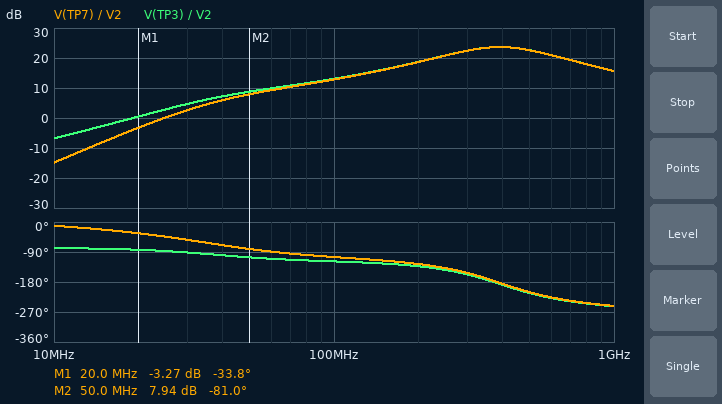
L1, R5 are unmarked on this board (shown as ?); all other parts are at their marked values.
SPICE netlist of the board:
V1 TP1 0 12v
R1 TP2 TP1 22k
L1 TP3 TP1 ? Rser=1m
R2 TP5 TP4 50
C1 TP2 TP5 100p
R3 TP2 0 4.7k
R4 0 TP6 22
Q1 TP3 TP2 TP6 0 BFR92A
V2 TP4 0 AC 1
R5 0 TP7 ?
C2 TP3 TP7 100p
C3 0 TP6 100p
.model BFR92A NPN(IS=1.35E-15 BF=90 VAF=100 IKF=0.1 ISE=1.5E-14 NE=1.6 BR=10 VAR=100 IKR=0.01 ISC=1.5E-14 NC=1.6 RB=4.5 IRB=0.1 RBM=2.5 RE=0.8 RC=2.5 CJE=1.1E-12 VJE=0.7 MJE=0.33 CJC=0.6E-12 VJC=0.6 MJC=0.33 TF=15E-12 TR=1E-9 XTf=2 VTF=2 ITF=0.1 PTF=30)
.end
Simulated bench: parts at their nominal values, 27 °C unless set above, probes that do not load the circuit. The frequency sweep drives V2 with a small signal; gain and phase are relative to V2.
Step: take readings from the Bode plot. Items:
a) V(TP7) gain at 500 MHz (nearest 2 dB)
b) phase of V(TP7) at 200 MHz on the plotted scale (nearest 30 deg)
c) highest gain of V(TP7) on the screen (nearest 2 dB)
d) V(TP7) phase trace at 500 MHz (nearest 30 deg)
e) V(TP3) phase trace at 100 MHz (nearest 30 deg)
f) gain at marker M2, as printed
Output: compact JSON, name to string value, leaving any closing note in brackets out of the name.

{"V(TP7) gain at 500 MHz": "22 dB", "phase of V(TP7) at 200 MHz on the plotted scale": "-120 deg", "highest gain of V(TP7) on the screen": "24 dB", "V(TP7) phase trace at 500 MHz": "-210 deg", "V(TP3) phase trace at 100 MHz": "-120 deg", "gain at marker M2, as printed": "7.94 dB"}
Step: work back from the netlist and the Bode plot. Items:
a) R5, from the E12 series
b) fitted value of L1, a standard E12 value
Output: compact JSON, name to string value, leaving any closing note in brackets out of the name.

{"R5, from the E12 series": "68 Ω", "fitted value of L1, a standard E12 value": "180 nH"}
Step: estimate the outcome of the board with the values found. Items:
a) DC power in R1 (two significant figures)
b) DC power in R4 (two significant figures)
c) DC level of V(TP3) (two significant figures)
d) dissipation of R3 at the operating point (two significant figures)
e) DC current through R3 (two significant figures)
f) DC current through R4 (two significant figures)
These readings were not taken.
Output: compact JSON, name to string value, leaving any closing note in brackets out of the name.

{"DC power in R1": "5.3 mW", "DC power in R4": "8.2 mW", "DC level of V(TP3)": "12 V", "dissipation of R3 at the operating point": "320 µW", "DC current through R3": "260 µA", "DC current through R4": "19 mA"}
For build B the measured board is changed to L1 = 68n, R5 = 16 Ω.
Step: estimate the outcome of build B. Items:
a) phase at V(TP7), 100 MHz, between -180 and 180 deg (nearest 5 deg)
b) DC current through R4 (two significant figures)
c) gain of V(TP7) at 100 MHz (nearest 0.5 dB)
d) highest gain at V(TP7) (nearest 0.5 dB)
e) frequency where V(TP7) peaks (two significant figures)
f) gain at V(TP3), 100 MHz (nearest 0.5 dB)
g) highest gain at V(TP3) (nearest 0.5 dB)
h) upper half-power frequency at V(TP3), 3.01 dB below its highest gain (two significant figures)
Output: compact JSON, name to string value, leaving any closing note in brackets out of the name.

{"phase at V(TP7), 100 MHz, between -180 and 180 deg": "-110 deg", "DC current through R4": "19 mA", "gain of V(TP7) at 100 MHz": "3.0 dB", "highest gain at V(TP7)": "11.5 dB", "frequency where V(TP7) peaks": "480 MHz", "gain at V(TP3), 100 MHz": "6.0 dB", "highest gain at V(TP3)": "12.0 dB", "upper half-power frequency at V(TP3), 3.01 dB below its highest gain": "810 MHz"}
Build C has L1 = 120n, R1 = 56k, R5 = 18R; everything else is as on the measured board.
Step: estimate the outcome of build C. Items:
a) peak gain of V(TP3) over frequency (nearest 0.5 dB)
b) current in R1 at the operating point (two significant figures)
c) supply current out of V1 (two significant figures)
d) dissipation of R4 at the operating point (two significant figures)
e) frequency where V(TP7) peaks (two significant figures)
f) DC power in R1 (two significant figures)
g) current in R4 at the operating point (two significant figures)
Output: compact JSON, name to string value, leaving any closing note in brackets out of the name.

{"peak gain of V(TP3) over frequency": "8.5 dB", "current in R1 at the operating point": "200 µA", "supply current out of V1": "3.1 mA", "dissipation of R4 at the operating point": "180 µW", "frequency where V(TP7) peaks": "400 MHz", "DC power in R1": "2.2 mW", "current in R4 at the operating point": "2.9 mA"}
